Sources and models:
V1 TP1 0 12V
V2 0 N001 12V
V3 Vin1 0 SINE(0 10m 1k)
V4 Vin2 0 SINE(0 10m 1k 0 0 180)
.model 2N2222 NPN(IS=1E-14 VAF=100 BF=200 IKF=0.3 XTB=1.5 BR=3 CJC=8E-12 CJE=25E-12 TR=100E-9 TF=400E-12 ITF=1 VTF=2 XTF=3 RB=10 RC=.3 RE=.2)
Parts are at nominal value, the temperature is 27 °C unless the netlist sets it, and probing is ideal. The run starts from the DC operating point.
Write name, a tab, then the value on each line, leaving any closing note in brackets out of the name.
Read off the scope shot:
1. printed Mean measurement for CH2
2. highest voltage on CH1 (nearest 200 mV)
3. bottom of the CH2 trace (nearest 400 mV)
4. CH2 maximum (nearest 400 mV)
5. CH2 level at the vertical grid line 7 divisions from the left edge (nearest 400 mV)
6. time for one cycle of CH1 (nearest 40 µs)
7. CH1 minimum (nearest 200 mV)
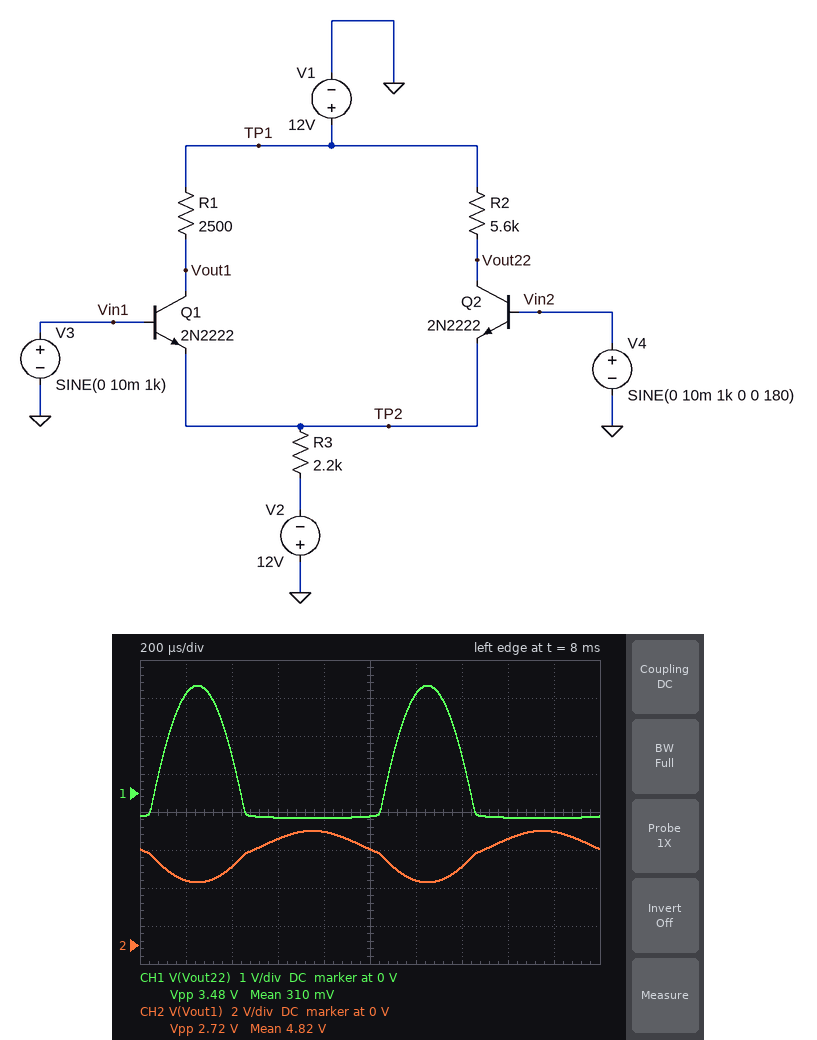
printed Mean measurement for CH2	4.82 V
highest voltage on CH1	2.8 V
bottom of the CH2 trace	3.2 V
CH2 maximum	6.0 V
CH2 level at the vertical grid line 7 divisions from the left edge	4.0 V
time for one cycle of CH1	1.00 ms
CH1 minimum	-600 mV
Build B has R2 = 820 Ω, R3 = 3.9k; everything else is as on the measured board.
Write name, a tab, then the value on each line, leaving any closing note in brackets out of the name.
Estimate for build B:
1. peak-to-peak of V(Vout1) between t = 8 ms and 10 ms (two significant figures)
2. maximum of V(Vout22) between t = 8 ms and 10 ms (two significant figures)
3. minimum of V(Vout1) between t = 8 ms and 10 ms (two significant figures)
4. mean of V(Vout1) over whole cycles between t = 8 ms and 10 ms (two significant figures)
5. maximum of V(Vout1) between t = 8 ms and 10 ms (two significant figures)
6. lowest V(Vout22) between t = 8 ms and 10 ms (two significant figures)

peak-to-peak of V(Vout1) between t = 8 ms and 10 ms	2.6 V
maximum of V(Vout22) between t = 8 ms and 10 ms	11 V
minimum of V(Vout1) between t = 8 ms and 10 ms	7.1 V
mean of V(Vout1) over whole cycles between t = 8 ms and 10 ms	8.4 V
maximum of V(Vout1) between t = 8 ms and 10 ms	9.7 V
lowest V(Vout22) between t = 8 ms and 10 ms	10 V
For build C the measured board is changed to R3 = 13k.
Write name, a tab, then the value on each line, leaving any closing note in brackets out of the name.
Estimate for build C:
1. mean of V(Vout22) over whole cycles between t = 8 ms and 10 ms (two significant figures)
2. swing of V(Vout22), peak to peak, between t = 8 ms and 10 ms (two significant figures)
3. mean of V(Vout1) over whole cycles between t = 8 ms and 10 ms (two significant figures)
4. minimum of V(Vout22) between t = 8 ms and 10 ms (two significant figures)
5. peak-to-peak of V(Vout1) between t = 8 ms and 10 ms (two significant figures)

mean of V(Vout22) over whole cycles between t = 8 ms and 10 ms	9.6 V
swing of V(Vout22), peak to peak, between t = 8 ms and 10 ms	1.8 V
mean of V(Vout1) over whole cycles between t = 8 ms and 10 ms	11 V
minimum of V(Vout22) between t = 8 ms and 10 ms	8.7 V
peak-to-peak of V(Vout1) between t = 8 ms and 10 ms	790 mV
